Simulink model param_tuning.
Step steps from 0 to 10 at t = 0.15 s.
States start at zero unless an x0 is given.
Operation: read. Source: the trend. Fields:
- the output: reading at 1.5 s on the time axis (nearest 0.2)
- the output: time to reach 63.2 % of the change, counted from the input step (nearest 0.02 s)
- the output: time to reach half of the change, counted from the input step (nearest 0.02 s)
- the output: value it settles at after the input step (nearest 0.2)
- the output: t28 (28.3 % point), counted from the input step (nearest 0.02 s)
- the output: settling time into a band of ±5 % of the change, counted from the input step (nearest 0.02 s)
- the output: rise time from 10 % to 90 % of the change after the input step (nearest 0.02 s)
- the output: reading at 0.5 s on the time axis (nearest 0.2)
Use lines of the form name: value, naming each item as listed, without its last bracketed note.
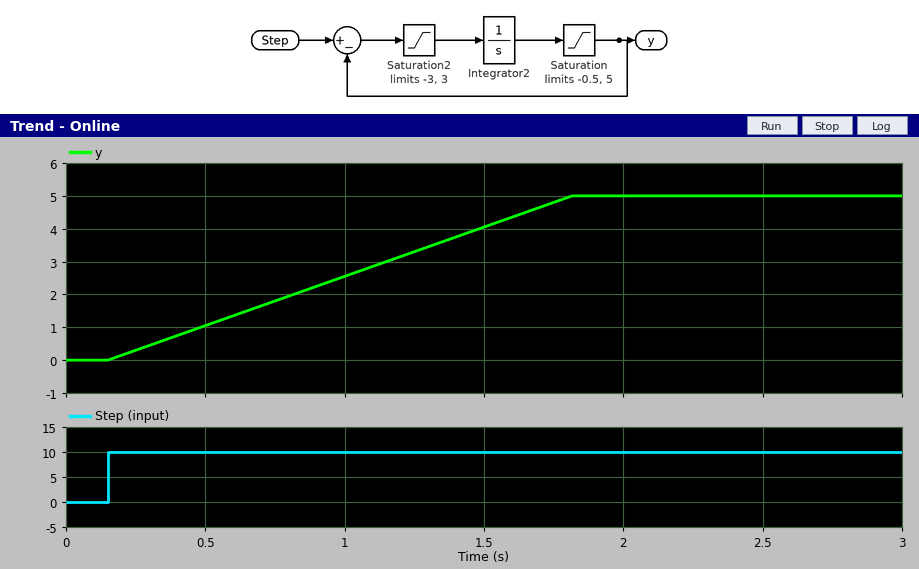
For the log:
the output: reading at 1.5 s on the time axis: 4.0
the output: time to reach 63.2 % of the change, counted from the input step: 1.06 s
the output: time to reach half of the change, counted from the input step: 0.84 s
the output: value it settles at after the input step: 5.0
the output: t28 (28.3 % point), counted from the input step: 0.48 s
the output: settling time into a band of ±5 % of the change, counted from the input step: 1.58 s
the output: rise time from 10 % to 90 % of the change after the input step: 1.34 s
the output: reading at 0.5 s on the time axis: 1.0
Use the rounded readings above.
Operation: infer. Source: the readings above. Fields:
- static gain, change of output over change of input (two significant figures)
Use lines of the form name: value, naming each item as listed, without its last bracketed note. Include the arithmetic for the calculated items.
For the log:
static gain, change of output over change of input: (5 - 0) / (10 - 0) = 0.50
